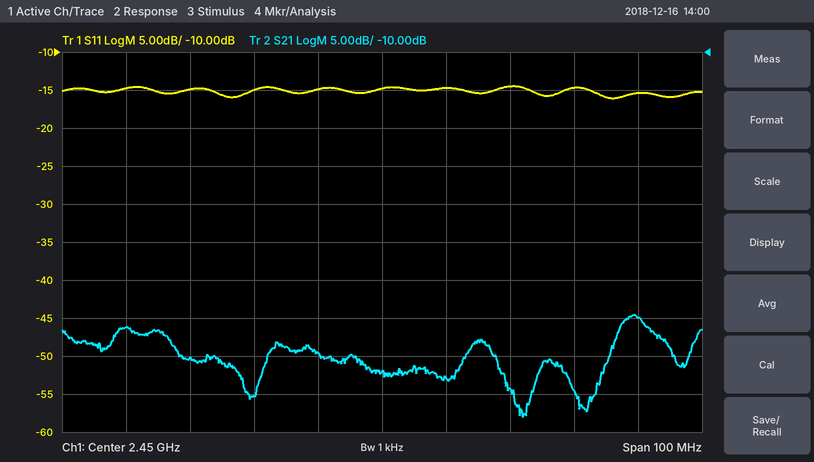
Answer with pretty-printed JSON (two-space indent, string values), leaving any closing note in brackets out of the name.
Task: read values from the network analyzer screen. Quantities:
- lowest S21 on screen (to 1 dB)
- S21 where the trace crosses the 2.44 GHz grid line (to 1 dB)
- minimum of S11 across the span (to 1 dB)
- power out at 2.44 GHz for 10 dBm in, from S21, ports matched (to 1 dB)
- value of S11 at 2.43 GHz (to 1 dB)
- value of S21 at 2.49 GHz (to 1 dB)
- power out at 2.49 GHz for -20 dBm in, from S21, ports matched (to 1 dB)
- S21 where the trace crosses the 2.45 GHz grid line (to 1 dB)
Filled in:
{
  "lowest S21 on screen": "-58 dB",
  "S21 where the trace crosses the 2.44 GHz grid line": "-50 dB",
  "minimum of S11 across the span": "-16 dB",
  "power out at 2.44 GHz for 10 dBm in, from S21, ports matched": "-40 dBm",
  "value of S11 at 2.43 GHz": "-15 dB",
  "value of S21 at 2.49 GHz": "-45 dB",
  "power out at 2.49 GHz for -20 dBm in, from S21, ports matched": "-65 dBm",
  "S21 where the trace crosses the 2.45 GHz grid line": "-52 dB"
}
